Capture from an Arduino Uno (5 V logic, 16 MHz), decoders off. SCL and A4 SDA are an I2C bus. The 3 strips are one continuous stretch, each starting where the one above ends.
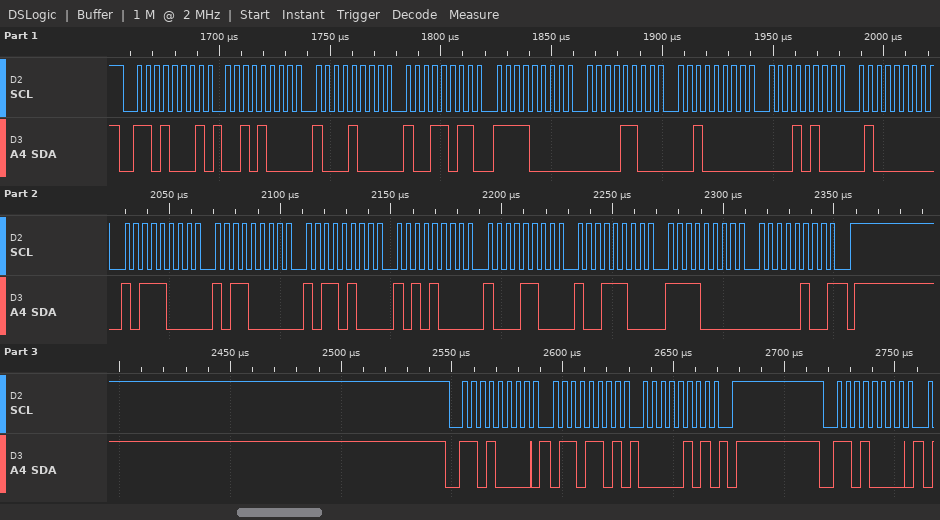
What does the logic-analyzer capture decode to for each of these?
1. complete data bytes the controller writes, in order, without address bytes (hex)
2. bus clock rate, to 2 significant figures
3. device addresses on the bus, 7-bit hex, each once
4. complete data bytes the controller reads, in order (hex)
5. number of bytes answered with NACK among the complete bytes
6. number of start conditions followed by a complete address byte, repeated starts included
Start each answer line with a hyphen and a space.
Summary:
- 6D 05
- 250 kHz
- 0x68
- 28 88 9B F0 0C 20 14 40 B8 B0 B4 A8 8C 9C F0 04
- 1
- 3
